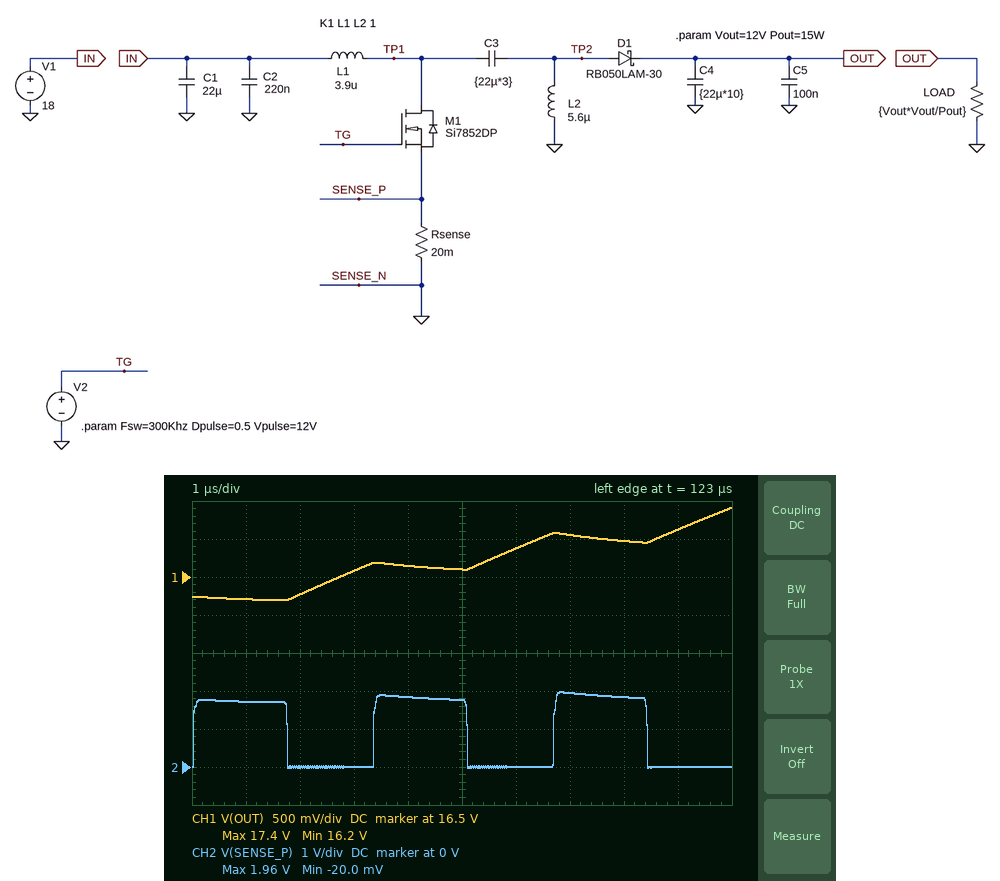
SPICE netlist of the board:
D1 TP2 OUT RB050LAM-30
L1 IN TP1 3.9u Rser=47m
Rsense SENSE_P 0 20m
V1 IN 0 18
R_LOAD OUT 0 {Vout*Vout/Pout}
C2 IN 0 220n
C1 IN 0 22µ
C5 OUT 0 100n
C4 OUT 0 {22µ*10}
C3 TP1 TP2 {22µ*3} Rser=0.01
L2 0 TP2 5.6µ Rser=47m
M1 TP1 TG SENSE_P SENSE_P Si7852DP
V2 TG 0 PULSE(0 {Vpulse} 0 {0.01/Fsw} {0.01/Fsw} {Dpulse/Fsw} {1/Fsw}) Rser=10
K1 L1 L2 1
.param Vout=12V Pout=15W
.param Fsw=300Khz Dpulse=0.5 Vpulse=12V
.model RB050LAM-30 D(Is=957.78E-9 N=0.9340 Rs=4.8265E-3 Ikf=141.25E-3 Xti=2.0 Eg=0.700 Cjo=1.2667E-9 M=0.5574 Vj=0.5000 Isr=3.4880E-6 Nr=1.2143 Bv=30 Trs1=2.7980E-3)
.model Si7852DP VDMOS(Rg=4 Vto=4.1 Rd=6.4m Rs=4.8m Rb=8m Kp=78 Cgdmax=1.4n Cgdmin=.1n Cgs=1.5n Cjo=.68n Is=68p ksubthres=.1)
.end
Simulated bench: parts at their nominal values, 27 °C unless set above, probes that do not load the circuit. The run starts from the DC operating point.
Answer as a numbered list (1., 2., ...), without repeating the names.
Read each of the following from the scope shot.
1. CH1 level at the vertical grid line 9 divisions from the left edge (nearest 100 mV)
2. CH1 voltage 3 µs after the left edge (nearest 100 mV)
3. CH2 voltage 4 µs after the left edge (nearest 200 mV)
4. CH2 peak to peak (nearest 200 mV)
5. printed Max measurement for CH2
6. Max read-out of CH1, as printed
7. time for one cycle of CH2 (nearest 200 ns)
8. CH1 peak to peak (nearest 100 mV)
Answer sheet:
1. 17.1 V
2. 16.6 V
3. 1.8 V
4. 2.0 V
5. 1.96 V
6. 17.4 V
7. 3.4 µs
8. 1.2 V
